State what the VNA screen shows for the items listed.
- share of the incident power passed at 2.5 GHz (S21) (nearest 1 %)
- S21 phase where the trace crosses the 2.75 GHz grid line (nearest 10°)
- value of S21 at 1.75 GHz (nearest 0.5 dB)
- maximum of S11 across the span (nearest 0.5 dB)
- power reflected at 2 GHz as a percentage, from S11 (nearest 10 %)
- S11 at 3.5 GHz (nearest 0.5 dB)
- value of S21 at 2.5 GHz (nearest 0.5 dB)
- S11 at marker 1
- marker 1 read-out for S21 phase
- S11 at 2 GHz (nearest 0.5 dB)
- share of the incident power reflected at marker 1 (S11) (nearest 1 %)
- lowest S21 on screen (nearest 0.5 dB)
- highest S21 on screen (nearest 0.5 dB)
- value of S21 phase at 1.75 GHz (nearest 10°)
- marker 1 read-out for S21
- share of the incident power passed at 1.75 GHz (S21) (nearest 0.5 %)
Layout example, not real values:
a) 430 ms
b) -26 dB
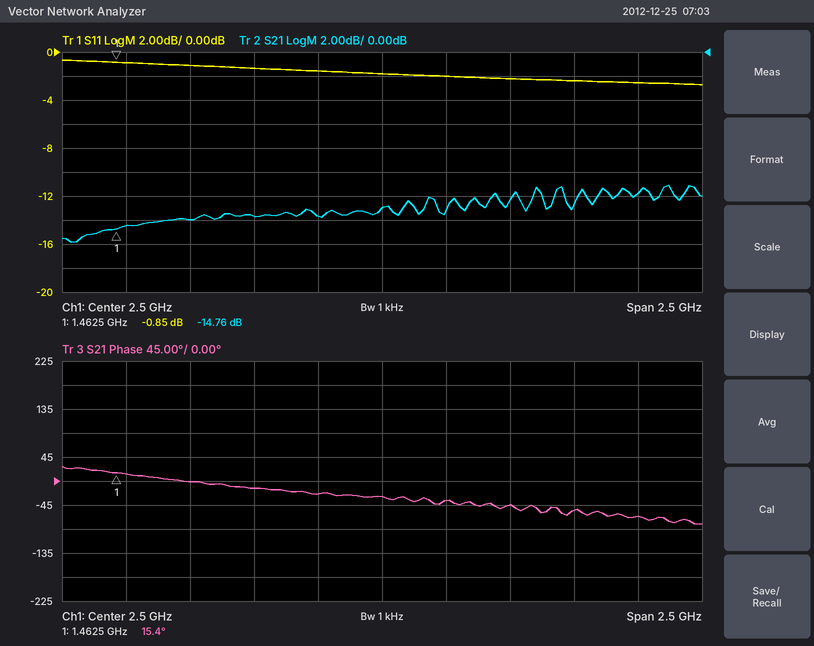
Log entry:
a) 5 %
b) -40°
c) -14.0 dB
d) -0.5 dB
e) 70 %
f) -2.5 dB
g) -13.0 dB
h) -0.85 dB
i) 15.4°
j) -1.5 dB
k) 82 %
l) -16.0 dB
m) -11.0 dB
n) 0°
o) -14.76 dB
p) 4.0 %
